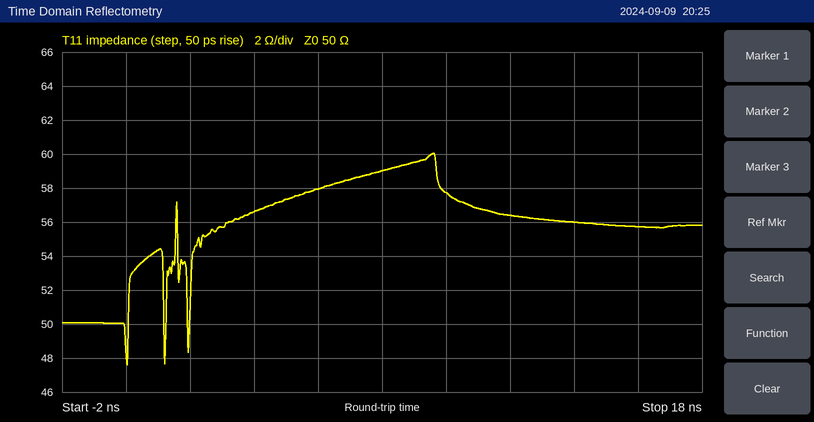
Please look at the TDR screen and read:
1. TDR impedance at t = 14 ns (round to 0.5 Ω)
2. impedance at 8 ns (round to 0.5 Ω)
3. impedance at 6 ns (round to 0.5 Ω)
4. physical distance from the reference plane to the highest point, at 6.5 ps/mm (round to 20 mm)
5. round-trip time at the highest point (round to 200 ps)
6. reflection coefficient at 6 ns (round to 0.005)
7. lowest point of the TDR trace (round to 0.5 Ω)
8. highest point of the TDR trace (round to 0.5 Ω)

56.0 Ω
59.0 Ω
58.0 Ω
740 mm
9.6 ns
+0.075
47.5 Ω
60.0 Ω
